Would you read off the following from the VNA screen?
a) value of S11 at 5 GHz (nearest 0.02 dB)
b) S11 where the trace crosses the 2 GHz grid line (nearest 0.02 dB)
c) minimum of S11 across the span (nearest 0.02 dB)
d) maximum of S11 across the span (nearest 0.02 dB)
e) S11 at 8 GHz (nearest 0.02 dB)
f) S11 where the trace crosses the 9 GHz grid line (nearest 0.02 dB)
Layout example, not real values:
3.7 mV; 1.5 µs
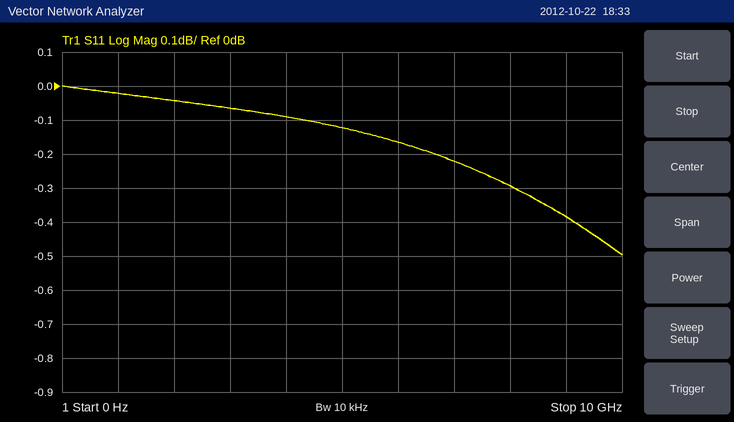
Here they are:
-0.12 dB; -0.04 dB; -0.50 dB; 0.00 dB; -0.30 dB; -0.38 dB
